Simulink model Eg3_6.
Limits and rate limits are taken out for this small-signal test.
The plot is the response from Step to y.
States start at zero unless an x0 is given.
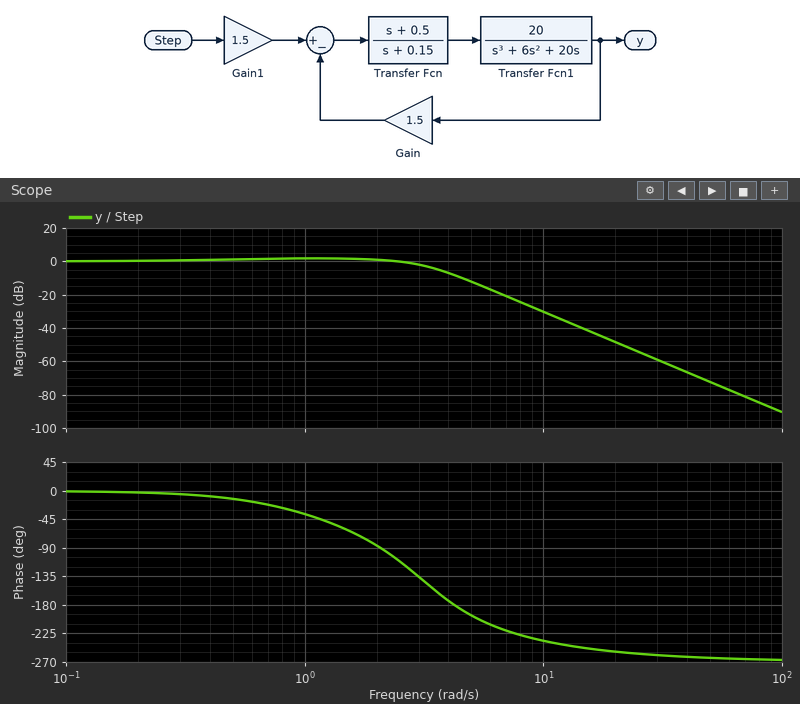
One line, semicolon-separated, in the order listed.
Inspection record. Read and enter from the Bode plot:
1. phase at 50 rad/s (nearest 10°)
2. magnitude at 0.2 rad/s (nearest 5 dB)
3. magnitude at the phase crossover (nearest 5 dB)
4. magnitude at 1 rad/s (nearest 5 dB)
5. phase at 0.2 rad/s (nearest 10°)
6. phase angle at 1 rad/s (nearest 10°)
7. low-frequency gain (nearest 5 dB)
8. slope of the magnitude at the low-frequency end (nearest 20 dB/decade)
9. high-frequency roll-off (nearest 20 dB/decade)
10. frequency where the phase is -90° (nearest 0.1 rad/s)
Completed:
-260°; 0 dB; -10 dB; 0 dB; 0°; -40°; 0 dB; 0 dB/decade; -60 dB/decade; 2.1 rad/s
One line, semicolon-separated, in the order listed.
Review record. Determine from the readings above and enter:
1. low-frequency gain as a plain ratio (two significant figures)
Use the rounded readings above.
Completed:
1.0
